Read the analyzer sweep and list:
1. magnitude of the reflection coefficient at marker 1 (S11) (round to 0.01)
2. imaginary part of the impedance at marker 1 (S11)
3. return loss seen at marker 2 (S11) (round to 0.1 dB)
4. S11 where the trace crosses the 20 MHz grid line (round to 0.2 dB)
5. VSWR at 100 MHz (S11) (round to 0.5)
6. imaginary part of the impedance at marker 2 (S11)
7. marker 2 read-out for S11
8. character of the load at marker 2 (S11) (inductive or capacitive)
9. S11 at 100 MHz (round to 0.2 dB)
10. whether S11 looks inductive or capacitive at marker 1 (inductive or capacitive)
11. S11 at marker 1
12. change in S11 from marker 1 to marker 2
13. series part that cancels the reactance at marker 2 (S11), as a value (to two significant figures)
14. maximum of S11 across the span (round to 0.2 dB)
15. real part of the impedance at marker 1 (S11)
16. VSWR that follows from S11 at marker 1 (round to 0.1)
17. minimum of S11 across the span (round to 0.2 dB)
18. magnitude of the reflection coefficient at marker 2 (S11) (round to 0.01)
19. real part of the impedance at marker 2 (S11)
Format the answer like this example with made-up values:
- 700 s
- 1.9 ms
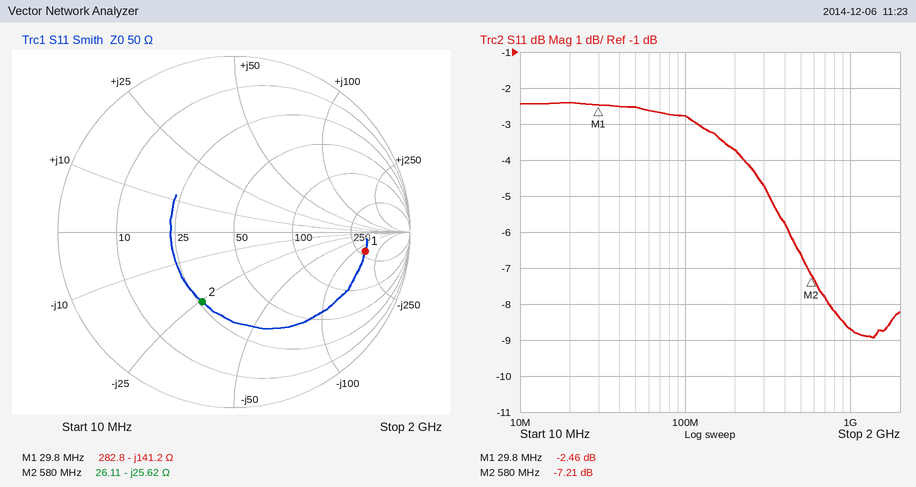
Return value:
- 0.75
- -141.2 Ω
- 7.2 dB
- -2.4 dB
- 6.5
- -25.62 Ω
- -7.21 dB
- capacitive
- -2.8 dB
- capacitive
- -2.46 dB
- -4.75 dB
- 7.0 nH
- -2.4 dB
- 282.8 Ω
- 7.1
- -9.0 dB
- 0.44
- 26.11 Ω
